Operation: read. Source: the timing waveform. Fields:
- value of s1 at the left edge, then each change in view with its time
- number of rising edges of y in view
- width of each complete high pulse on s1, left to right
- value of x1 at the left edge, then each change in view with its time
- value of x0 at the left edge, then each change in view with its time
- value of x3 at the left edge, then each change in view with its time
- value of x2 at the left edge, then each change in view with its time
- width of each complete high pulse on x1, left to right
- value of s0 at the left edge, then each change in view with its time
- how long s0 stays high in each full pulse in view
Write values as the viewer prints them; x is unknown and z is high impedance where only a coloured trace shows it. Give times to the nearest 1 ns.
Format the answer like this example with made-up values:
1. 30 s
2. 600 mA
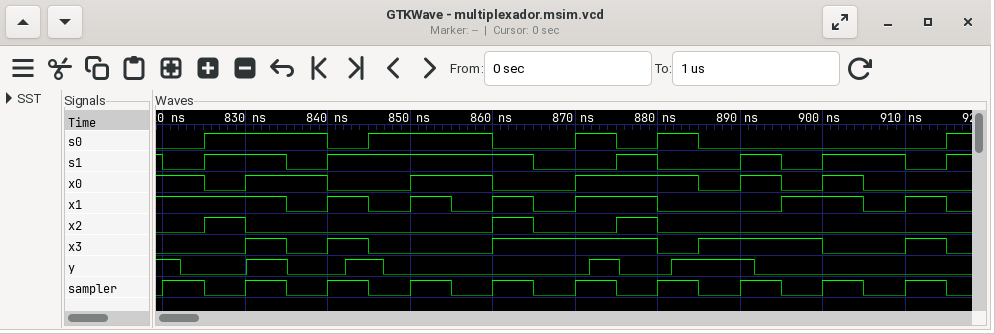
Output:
1. 1, 0 at 820 ns, 1 at 825 ns, 0 at 835 ns, 1 at 840 ns, 0 at 865 ns, 1 at 875 ns, 0 at 880 ns, 1 at 890 ns, 0 at 895 ns, 1 at 900 ns, 0 at 910 ns, 1 at 915 ns
2. 4
3. 10 ns, 25 ns, 5 ns, 5 ns, 10 ns
4. 1, 0 at 835 ns, 1 at 840 ns, 0 at 845 ns, 1 at 850 ns, 0 at 855 ns, 1 at 860 ns, 0 at 865 ns, 1 at 870 ns, 0 at 880 ns, 1 at 895 ns, 0 at 905 ns, 1 at 910 ns, 0 at 915 ns
5. 1, 0 at 825 ns, 1 at 830 ns, 0 at 840 ns, 1 at 850 ns, 0 at 860 ns, 1 at 870 ns, 0 at 885 ns, 1 at 890 ns, 0 at 895 ns, 1 at 900 ns, 0 at 905 ns
6. 0, 1 at 830 ns, 0 at 835 ns, 1 at 840 ns, 0 at 845 ns, 1 at 860 ns, 0 at 880 ns, 1 at 885 ns, 0 at 900 ns, 1 at 910 ns, 0 at 915 ns
7. 0, 1 at 825 ns, 0 at 830 ns, 1 at 860 ns, 0 at 865 ns, 1 at 875 ns, 0 at 880 ns
8. 5 ns, 5 ns, 5 ns, 10 ns, 10 ns, 5 ns
9. 0, 1 at 825 ns, 0 at 840 ns, 1 at 845 ns, 0 at 860 ns, 1 at 870 ns, 0 at 875 ns, 1 at 880 ns, 0 at 885 ns, 1 at 915 ns
10. 15 ns, 15 ns, 5 ns, 5 ns
